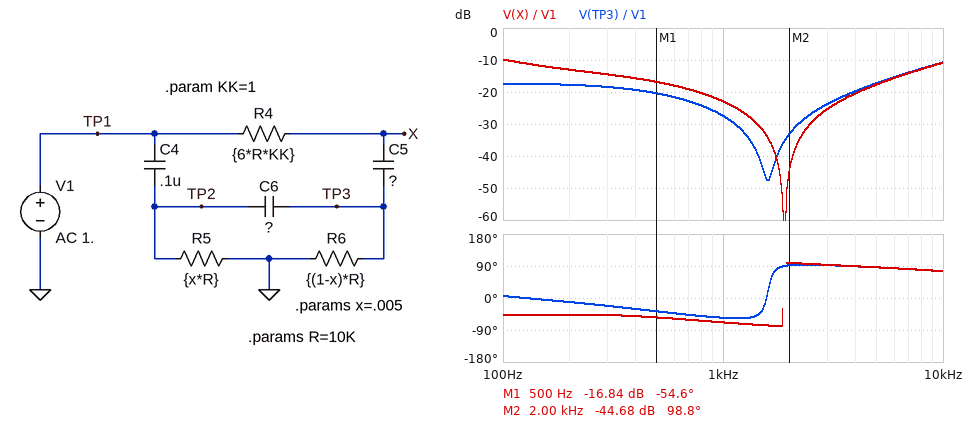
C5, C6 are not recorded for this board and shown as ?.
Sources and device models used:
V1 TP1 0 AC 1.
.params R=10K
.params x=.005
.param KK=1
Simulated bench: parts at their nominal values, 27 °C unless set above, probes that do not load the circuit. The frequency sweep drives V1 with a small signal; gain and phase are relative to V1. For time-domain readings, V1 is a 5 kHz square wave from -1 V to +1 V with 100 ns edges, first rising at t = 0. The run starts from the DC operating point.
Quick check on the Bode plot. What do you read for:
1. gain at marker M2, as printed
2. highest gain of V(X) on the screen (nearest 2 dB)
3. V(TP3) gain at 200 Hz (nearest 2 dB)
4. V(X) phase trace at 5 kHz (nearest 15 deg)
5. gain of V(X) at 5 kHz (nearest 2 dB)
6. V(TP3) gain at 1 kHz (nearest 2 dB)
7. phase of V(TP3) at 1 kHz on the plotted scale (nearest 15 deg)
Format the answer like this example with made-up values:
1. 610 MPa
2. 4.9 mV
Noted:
1. -44.68 dB
2. -10 dB
3. -18 dB
4. 90 deg
5. -18 dB
6. -28 dB
7. -60 deg
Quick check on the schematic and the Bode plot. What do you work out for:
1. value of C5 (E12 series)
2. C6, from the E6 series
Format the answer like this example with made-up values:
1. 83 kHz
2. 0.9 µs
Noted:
1. 82 nF
2. 33 nF
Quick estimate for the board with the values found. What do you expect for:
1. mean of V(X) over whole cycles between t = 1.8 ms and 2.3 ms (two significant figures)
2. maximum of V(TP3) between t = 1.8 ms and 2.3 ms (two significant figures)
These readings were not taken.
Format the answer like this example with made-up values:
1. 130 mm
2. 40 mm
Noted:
1. -590 mV
2. 2.1 V
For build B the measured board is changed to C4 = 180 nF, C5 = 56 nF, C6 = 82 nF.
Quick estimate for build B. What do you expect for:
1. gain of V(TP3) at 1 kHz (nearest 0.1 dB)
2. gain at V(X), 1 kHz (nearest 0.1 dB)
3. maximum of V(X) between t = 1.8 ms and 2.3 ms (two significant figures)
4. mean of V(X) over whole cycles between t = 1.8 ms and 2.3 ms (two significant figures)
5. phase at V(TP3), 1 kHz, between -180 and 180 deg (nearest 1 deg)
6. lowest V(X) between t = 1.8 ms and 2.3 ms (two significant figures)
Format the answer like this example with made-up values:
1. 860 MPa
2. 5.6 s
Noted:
1. -32.4 dB
2. -32.6 dB
3. 1.5 V
4. -460 mV
5. 90 deg
6. -2.5 V
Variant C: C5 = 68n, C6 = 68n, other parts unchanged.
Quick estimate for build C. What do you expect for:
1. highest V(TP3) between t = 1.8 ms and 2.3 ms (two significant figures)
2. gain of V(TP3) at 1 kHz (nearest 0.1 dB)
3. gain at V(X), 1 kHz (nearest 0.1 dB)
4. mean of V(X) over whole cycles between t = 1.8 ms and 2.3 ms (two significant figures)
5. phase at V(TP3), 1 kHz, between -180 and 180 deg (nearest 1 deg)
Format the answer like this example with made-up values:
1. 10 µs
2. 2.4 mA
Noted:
1. 2.1 V
2. -42.0 dB
3. -26.9 dB
4. -520 mV
5. -51 deg
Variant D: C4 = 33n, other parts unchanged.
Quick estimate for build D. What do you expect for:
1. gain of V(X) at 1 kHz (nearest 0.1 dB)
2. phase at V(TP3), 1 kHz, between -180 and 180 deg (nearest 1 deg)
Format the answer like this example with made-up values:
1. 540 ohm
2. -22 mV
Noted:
1. -21.0 dB
2. -58 deg
